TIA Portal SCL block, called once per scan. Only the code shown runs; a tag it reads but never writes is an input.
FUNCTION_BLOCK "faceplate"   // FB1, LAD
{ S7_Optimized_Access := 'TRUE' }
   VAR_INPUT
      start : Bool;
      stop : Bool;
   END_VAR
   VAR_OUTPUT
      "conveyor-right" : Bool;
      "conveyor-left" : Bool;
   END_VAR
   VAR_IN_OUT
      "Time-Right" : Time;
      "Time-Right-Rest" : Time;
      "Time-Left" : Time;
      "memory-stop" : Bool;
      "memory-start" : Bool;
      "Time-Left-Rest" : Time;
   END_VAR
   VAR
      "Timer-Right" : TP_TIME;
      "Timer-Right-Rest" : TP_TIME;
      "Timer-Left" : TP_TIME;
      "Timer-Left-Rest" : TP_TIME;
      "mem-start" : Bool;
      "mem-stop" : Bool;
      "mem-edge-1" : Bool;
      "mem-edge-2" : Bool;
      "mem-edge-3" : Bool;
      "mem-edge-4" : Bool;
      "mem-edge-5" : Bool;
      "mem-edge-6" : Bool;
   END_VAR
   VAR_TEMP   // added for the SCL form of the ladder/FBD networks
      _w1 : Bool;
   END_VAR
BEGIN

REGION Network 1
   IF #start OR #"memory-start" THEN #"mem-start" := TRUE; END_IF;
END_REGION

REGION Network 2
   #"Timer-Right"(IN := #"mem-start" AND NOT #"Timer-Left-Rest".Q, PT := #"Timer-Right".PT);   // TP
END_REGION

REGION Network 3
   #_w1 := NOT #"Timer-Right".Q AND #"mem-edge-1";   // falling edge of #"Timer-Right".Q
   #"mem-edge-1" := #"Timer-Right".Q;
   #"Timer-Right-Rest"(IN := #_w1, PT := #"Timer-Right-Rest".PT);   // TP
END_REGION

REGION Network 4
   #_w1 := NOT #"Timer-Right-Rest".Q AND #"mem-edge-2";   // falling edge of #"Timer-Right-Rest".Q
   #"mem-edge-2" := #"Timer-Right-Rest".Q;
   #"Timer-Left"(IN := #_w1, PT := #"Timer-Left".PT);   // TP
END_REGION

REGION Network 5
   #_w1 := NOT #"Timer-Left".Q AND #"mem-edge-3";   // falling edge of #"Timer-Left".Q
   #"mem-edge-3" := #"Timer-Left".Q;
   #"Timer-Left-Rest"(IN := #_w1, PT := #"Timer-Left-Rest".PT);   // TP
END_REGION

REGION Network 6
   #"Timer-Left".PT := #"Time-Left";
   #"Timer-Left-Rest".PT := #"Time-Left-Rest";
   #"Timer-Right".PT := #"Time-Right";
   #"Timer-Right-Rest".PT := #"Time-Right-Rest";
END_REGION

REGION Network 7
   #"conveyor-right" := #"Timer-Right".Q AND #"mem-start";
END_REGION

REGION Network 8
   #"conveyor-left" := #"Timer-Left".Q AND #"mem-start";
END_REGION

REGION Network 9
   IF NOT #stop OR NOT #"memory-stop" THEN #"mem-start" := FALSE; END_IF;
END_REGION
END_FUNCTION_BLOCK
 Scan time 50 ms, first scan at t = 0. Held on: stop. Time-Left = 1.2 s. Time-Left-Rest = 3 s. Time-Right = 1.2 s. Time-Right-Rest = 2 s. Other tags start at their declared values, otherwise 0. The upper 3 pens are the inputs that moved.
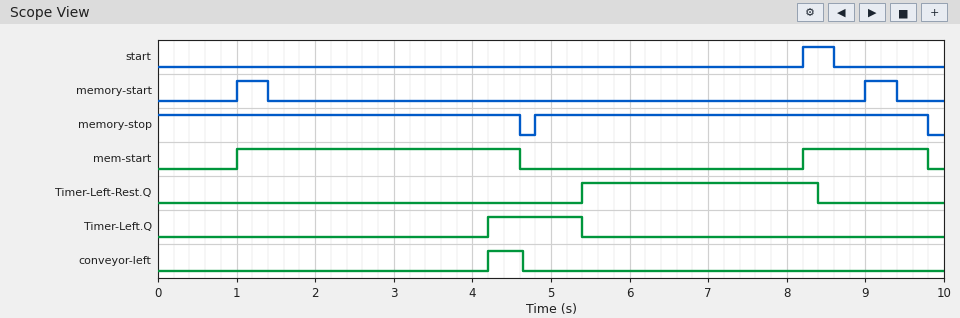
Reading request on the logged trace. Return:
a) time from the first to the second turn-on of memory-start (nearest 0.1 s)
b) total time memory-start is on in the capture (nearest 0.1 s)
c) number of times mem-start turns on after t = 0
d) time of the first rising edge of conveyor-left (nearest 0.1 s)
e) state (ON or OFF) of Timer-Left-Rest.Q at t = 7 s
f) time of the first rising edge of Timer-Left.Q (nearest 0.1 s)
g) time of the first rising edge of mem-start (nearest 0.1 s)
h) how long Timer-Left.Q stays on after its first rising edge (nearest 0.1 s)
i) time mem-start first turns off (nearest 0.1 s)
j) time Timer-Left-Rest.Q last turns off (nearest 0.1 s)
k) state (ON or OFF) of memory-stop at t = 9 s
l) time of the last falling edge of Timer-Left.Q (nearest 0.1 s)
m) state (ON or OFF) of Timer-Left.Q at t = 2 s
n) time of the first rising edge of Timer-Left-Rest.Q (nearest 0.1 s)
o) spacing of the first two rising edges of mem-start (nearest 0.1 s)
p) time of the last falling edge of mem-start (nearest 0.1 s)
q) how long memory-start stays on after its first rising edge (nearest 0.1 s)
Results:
8.0 s
0.8 s
2
4.2 s
ON
4.2 s
1.0 s
1.2 s
4.6 s
8.4 s
ON
5.4 s
OFF
5.4 s
7.2 s
9.8 s
0.4 s
